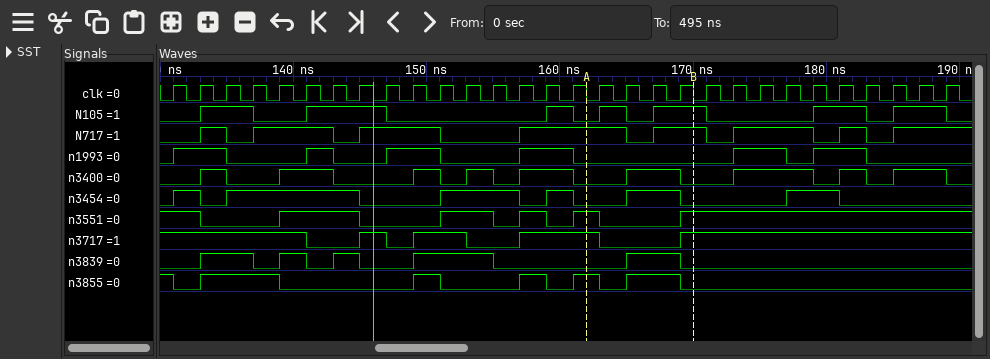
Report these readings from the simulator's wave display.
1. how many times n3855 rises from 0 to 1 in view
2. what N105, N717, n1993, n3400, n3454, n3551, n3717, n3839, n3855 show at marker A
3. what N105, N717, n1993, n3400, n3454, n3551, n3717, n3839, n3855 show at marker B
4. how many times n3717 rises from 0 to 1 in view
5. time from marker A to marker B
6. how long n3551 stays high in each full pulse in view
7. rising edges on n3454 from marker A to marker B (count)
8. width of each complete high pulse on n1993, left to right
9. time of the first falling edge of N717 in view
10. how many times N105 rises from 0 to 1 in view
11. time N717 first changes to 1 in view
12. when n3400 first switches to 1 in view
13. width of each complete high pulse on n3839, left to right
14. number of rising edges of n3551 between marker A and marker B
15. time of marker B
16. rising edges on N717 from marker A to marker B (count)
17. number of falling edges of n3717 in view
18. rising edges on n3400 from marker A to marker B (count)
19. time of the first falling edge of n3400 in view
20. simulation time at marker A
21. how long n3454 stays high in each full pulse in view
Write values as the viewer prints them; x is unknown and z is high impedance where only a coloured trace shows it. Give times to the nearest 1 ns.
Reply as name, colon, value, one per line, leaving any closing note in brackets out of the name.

how many times n3855 rises from 0 to 1 in view: 5
what N105, N717, n1993, n3400, n3454, n3551, n3717, n3839, n3855 show at marker A: N105=0, N717=1, n1993=0, n3400=0, n3454=0, n3551=1, n3717=1, n3839=0, n3855=1
what N105, N717, n1993, n3400, n3454, n3551, n3717, n3839, n3855 show at marker B: N105=1, N717=1, n1993=0, n3400=0, n3454=0, n3551=1, n3717=1, n3839=0, n3855=0
how many times n3717 rises from 0 to 1 in view: 4
time from marker A to marker B: 8 ns
how long n3551 stays high in each full pulse in view: 6 ns, 4 ns, 2 ns, 2 ns
rising edges on n3454 from marker A to marker B: 1
width of each complete high pulse on n1993, left to right: 4 ns, 2 ns, 4 ns, 4 ns, 4 ns, 4 ns
time of the first falling edge of N717 in view: 135 ns
how many times N105 rises from 0 to 1 in view: 7
time N717 first changes to 1 in view: 133 ns
when n3400 first switches to 1 in view: 133 ns
width of each complete high pulse on n3839, left to right: 4 ns, 2 ns, 2 ns, 6 ns, 4 ns
number of rising edges of n3551 between marker A and marker B: 1
time of marker B: 170 ns
rising edges on N717 from marker A to marker B: 1
number of falling edges of n3717 in view: 4
rising edges on n3400 from marker A to marker B: 1
time of the first falling edge of n3400 in view: 135 ns
simulation time at marker A: 162 ns
how long n3454 stays high in each full pulse in view: 2 ns, 10 ns, 6 ns, 2 ns, 4 ns, 4 ns
